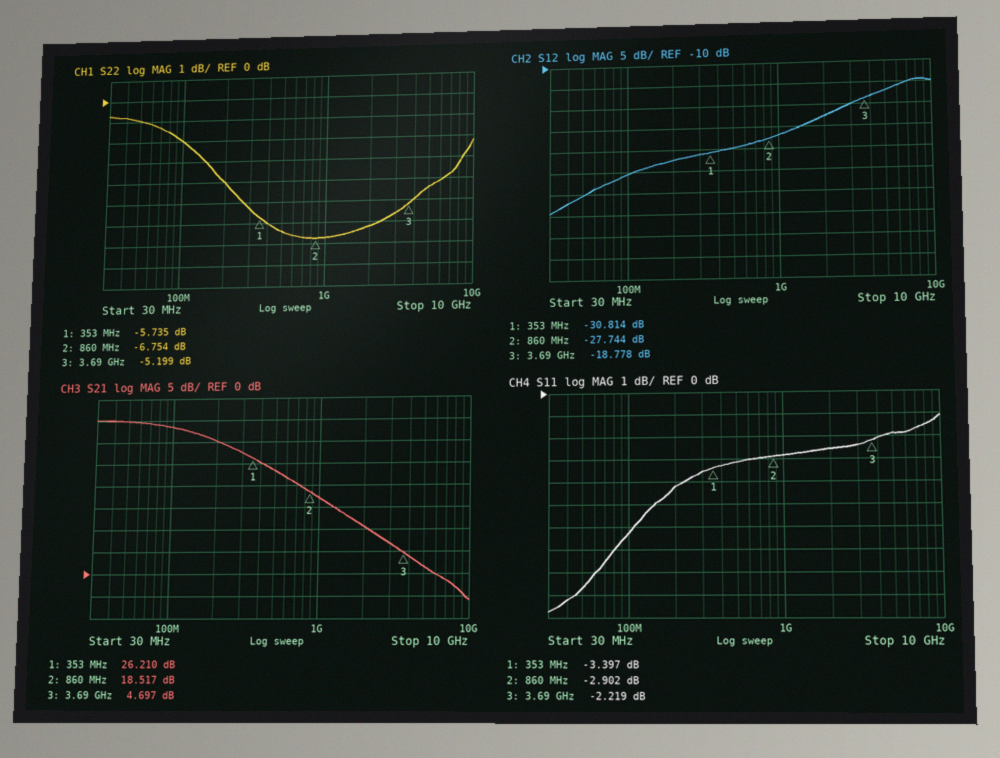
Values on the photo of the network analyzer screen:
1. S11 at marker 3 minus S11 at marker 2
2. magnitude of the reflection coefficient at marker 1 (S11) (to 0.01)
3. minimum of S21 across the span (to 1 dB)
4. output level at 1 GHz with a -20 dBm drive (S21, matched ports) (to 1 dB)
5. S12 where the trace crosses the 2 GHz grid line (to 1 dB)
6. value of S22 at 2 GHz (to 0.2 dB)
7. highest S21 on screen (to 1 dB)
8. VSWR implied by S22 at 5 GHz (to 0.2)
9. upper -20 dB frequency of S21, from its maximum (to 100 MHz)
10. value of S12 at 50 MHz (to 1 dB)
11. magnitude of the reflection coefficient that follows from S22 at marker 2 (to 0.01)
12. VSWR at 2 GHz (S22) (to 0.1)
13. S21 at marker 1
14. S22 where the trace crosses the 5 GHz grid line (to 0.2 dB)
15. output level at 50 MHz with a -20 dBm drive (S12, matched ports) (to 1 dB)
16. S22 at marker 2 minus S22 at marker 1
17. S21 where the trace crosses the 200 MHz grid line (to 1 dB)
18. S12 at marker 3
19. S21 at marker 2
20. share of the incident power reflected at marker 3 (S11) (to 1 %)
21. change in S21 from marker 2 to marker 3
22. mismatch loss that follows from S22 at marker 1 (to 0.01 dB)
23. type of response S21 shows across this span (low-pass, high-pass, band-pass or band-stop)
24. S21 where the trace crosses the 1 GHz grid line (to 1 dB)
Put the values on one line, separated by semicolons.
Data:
0.683 dB; 0.68; -6 dB; -3 dBm; -23 dB; -6.2 dB; 35 dB; 4.0; 1.2 GHz; -40 dB; 0.46; 2.9; 26.210 dB; -4.4 dB; -60 dBm; -1.019 dB; 30 dB; -18.778 dB; 18.517 dB; 60 %; -13.820 dB; 1.35 dB; low-pass; 17 dB
